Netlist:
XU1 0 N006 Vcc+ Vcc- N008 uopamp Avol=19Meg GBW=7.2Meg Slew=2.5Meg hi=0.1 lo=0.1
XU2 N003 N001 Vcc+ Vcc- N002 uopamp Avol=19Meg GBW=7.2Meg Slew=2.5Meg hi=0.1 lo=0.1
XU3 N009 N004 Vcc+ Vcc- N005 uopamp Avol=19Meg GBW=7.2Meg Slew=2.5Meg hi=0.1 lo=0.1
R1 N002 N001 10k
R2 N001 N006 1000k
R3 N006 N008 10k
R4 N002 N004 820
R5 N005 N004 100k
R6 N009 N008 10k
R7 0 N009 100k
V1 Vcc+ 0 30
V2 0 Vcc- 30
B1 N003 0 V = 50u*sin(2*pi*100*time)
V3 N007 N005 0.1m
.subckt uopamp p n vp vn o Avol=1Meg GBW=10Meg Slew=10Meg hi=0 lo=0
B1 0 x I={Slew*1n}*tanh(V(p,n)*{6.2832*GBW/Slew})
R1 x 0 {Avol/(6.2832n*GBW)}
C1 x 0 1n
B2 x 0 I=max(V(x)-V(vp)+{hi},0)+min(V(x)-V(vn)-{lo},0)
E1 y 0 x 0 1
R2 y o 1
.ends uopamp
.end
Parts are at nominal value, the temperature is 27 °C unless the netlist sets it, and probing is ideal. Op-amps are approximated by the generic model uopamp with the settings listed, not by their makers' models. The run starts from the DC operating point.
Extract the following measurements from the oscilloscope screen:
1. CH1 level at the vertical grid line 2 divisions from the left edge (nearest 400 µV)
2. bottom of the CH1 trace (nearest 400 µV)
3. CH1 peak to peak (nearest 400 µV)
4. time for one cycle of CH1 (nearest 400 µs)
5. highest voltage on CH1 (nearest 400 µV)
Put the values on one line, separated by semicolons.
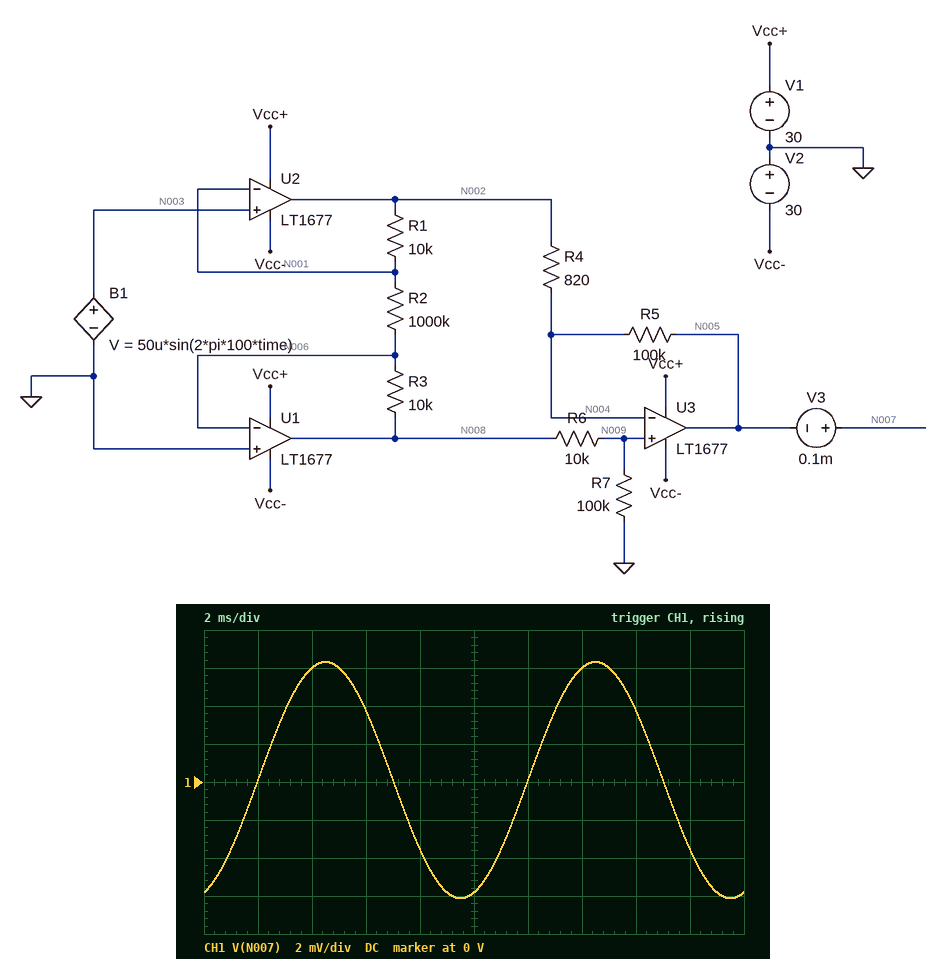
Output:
6.0 mV; -6.0 mV; 12.4 mV; 10.0 ms; 6.4 mV
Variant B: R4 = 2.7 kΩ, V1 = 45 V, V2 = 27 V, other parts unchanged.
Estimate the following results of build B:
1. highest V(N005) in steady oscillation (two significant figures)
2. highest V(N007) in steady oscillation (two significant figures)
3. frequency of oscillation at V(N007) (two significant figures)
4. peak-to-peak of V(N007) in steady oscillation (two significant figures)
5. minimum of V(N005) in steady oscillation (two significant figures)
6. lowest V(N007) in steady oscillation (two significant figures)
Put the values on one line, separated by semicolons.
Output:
1.9 mV; 2.0 mV; 100 Hz; 3.8 mV; -1.9 mV; -1.8 mV
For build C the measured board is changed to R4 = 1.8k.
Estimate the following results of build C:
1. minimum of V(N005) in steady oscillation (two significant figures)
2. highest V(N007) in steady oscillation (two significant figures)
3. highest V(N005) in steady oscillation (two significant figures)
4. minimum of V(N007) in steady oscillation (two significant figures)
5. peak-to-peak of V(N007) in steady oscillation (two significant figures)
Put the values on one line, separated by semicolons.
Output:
-2.8 mV; 2.9 mV; 2.8 mV; -2.7 mV; 5.7 mV
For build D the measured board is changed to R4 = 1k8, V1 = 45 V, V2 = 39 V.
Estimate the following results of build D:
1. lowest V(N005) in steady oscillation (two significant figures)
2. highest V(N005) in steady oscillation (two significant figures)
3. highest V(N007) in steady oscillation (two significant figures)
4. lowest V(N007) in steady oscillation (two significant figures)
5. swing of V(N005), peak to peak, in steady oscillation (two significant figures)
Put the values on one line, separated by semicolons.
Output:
-2.8 mV; 2.8 mV; 2.9 mV; -2.7 mV; 5.7 mV
